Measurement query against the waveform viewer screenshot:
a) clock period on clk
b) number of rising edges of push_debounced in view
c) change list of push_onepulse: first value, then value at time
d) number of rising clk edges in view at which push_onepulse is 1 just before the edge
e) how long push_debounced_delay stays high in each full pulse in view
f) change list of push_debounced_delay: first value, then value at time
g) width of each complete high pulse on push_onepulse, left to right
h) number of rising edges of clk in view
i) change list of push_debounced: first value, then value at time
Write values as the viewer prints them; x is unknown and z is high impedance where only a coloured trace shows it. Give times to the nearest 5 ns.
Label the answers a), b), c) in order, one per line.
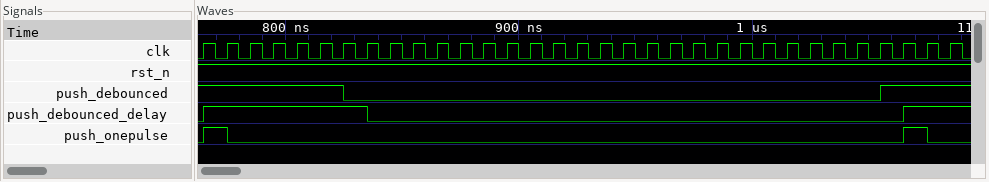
a) 10 ns
b) 1
c) 0, 1 at 765 ns, 0 at 775 ns, 1 at 1065 ns, 0 at 1075 ns
d) 2
e) 70 ns
f) 0, 1 at 765 ns, 0 at 835 ns, 1 at 1065 ns
g) 10 ns, 10 ns
h) 33
i) 1, 0 at 825 ns, 1 at 1055 ns
